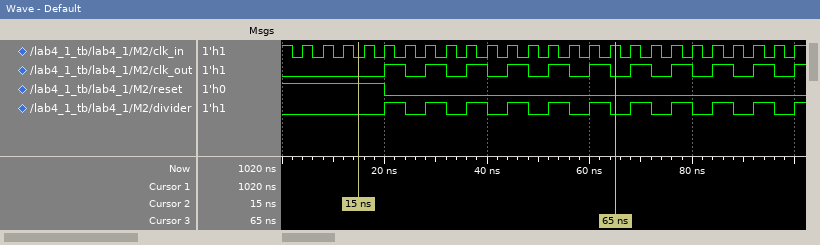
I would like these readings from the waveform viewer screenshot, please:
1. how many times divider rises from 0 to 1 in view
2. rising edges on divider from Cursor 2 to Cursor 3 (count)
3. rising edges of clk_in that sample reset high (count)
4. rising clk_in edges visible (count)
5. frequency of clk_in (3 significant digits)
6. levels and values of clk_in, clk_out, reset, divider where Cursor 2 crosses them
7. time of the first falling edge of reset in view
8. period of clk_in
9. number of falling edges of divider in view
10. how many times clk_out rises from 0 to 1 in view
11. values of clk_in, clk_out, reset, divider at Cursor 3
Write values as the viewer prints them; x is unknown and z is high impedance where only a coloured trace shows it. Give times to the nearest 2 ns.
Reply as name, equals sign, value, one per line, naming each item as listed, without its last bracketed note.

how many times divider rises from 0 to 1 in view = 11
rising edges on divider from Cursor 2 to Cursor 3 = 6
rising edges of clk_in that sample reset high = 5
rising clk_in edges visible = 25
frequency of clk_in = 250 MHz
levels and values of clk_in, clk_out, reset, divider where Cursor 2 crosses them = clk_in=0, clk_out=0, reset=1, divider=0
time of the first falling edge of reset in view = 20 ns
period of clk_in = 4 ns
number of falling edges of divider in view = 10
how many times clk_out rises from 0 to 1 in view = 11
values of clk_in, clk_out, reset, divider at Cursor 3 = clk_in=1, clk_out=0, reset=0, divider=0
